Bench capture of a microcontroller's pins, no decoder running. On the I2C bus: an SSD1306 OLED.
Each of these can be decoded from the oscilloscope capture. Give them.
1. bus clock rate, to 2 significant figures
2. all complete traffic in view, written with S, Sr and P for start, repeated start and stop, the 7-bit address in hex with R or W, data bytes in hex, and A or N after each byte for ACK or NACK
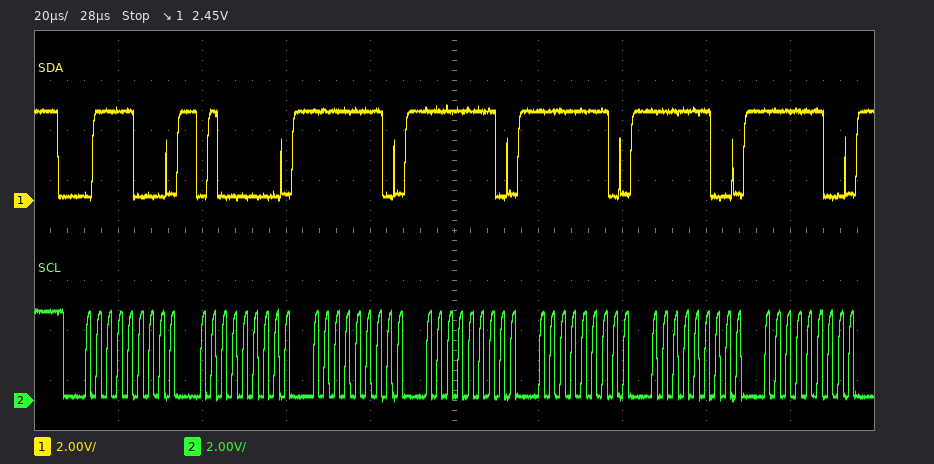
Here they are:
400 kHz
S 3CW A 40 A FE A FE A FE A FC A FC A
